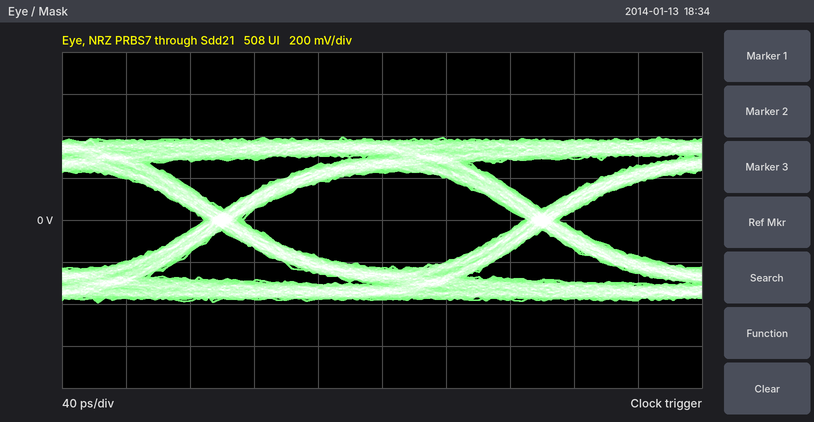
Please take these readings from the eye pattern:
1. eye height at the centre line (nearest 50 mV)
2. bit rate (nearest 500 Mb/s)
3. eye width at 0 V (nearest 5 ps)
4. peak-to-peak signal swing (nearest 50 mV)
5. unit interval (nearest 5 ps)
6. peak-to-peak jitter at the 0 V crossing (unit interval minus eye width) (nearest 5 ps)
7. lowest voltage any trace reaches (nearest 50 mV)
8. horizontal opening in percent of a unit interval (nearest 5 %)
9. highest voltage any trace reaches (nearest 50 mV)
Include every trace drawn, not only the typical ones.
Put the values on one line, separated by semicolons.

450 mV; 5.0 Gb/s; 175 ps; 800 mV; 200 ps; 25 ps; -400 mV; 90 %; 400 mV
